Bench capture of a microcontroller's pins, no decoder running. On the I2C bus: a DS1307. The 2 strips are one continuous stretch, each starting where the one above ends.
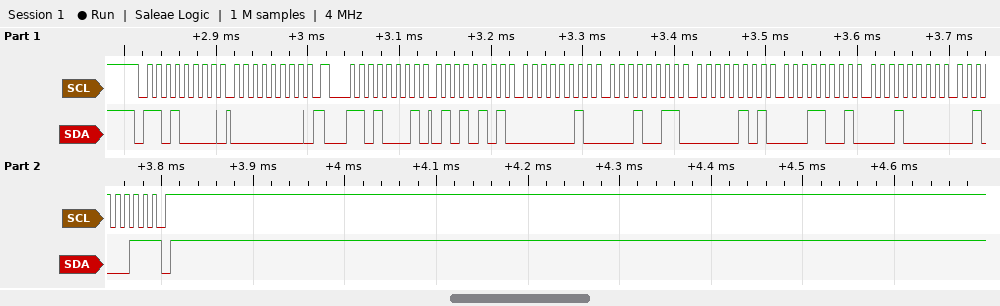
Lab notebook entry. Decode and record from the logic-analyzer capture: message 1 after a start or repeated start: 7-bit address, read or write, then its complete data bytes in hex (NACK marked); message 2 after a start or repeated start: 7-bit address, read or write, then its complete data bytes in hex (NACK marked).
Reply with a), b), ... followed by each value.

a) 0x68 write: 00
b) 0x68 read: 55 02 13 05 19 10 23 NACK
